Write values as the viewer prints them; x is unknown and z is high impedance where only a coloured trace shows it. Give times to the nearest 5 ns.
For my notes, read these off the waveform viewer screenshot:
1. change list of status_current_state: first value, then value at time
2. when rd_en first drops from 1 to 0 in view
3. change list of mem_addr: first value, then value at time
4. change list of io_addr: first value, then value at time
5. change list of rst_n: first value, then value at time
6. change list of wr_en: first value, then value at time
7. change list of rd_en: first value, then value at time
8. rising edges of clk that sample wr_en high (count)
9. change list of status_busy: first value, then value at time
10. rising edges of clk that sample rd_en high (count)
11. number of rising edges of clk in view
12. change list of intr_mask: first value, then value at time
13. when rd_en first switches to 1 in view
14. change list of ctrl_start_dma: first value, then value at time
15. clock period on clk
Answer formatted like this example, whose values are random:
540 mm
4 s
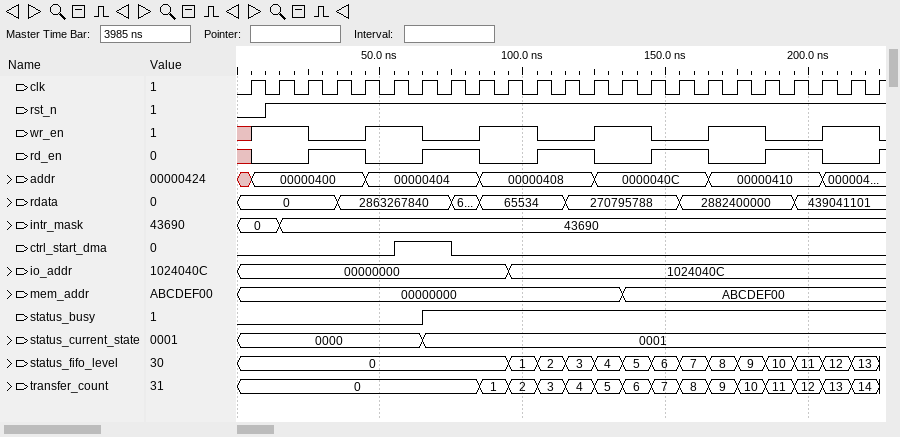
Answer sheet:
0000, 0001 at 65 ns
45 ns
00000000, ABCDEF00 at 135 ns
00000000, 1024040C at 95 ns
0, 1 at 10 ns
x, 1 at 5 ns, 0 at 25 ns, 1 at 45 ns, 0 at 65 ns, 1 at 85 ns, 0 at 105 ns, 1 at 125 ns, 0 at 145 ns, 1 at 165 ns, 0 at 185 ns, 1 at 205 ns, 0 at 225 ns
x, 0 at 5 ns, 1 at 25 ns, 0 at 45 ns, 1 at 65 ns, 0 at 85 ns, 1 at 105 ns, 0 at 125 ns, 1 at 145 ns, 0 at 165 ns, 1 at 185 ns, 0 at 205 ns, 1 at 225 ns
12
0, 1 at 65 ns
10
23
0, 43690 at 15 ns
25 ns
0, 1 at 55 ns, 0 at 75 ns
10 ns
